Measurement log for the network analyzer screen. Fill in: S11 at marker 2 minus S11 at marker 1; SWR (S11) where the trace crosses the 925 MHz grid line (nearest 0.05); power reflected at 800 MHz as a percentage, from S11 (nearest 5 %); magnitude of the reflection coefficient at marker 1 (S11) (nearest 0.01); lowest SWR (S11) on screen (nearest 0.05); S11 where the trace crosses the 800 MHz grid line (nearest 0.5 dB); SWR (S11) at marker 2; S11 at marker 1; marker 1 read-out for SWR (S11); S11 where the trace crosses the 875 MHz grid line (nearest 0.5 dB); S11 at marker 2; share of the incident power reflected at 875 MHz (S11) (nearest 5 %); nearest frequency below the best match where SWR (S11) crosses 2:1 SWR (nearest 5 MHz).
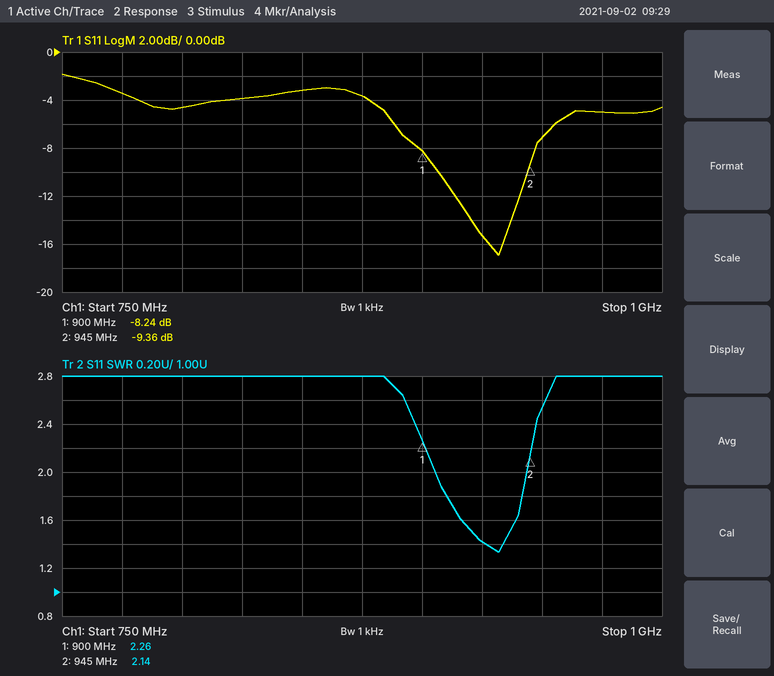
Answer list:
-1.12 dB
1.40
35 %
0.39
1.35
-4.5 dB
2.14
-8.24 dB
2.26
-3.5 dB
-9.36 dB
45 %
905 MHz
